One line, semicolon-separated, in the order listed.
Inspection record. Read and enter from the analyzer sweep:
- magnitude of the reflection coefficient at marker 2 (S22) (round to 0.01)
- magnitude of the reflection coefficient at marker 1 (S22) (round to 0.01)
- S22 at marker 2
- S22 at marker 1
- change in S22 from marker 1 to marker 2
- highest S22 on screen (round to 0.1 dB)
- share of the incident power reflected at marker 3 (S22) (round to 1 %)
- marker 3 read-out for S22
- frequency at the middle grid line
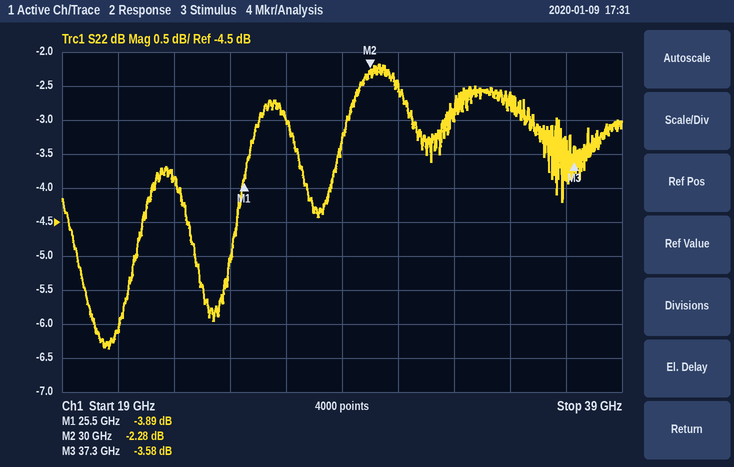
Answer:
0.77; 0.64; -2.28 dB; -3.89 dB; 1.61 dB; -2.2 dB; 44 %; -3.58 dB; 29 GHz
